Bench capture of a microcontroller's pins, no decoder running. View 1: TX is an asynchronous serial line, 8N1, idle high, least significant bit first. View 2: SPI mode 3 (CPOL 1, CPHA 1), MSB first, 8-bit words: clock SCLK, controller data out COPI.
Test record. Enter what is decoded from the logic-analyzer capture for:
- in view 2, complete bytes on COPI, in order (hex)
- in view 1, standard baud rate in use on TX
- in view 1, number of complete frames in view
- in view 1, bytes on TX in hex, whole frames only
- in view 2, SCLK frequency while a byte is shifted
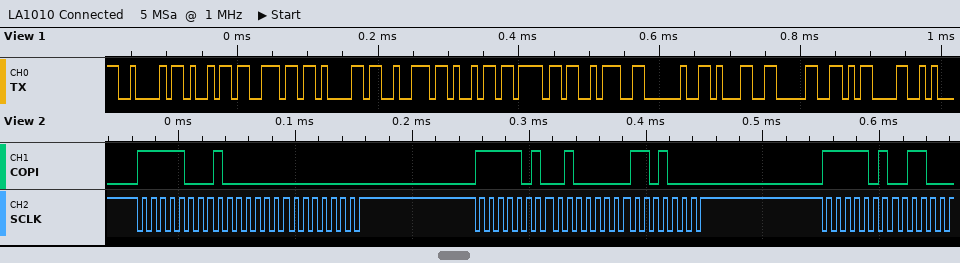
0xF8 0x80 0x00 0xFA 0x40 0xD0 0xFA
115200 baud
12
42 69 6E 61 72 69 6F 3A 20 31 30 0D
125 kHz
